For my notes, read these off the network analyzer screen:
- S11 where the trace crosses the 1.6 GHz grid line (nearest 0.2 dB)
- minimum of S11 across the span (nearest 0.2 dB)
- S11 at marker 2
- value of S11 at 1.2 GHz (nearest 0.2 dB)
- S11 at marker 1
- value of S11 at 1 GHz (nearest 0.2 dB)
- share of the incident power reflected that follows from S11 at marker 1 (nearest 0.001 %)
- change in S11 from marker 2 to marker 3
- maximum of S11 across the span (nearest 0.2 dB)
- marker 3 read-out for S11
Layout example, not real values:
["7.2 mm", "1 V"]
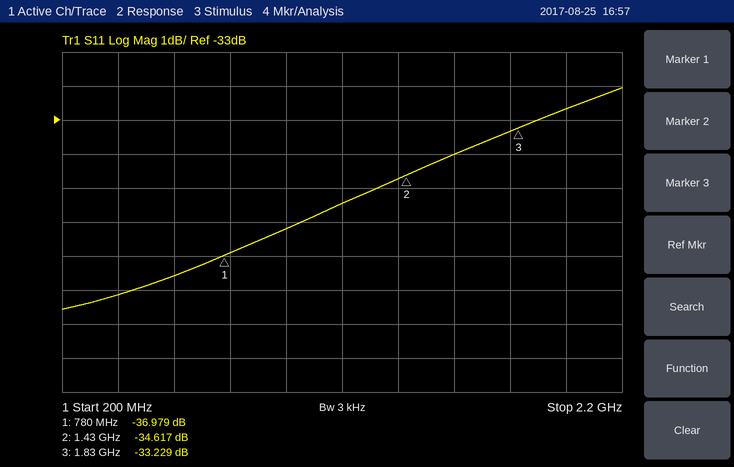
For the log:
["-34.0 dB", "-38.6 dB", "-34.617 dB", "-35.4 dB", "-36.979 dB", "-36.2 dB", "0.020 %", "1.388 dB", "-32.0 dB", "-33.229 dB"]
